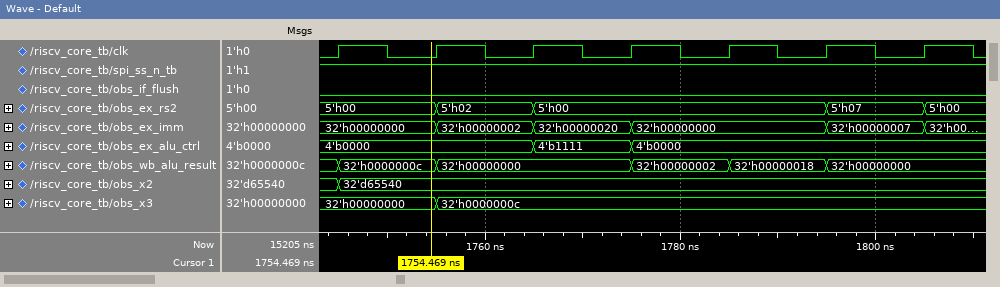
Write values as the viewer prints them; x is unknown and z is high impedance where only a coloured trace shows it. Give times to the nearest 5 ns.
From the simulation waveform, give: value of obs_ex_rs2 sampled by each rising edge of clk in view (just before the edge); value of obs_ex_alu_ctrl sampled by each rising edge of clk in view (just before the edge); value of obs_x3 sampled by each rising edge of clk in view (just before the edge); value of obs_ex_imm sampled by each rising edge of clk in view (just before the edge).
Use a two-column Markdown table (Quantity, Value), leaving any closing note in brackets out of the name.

| Quantity | Value |
|---|---|
| value of obs_ex_rs2 sampled by each rising edge of clk in view | 5'h00, 5'h00, 5'h02, 5'h00, 5'h00, 5'h00, 5'h07 |
| value of obs_ex_alu_ctrl sampled by each rising edge of clk in view | 4'b0000, 4'b0000, 4'b0000, 4'b1111, 4'b0000, 4'b0000, 4'b0000 |
| value of obs_x3 sampled by each rising edge of clk in view | 32'h00000000, 32'h00000000, 32'h0000000c, 32'h0000000c, 32'h0000000c, 32'h0000000c, 32'h0000000c |
| value of obs_ex_imm sampled by each rising edge of clk in view | 32'h00000000, 32'h00000000, 32'h00000002, 32'h00000020, 32'h00000000, 32'h00000000, 32'h00000007 |
